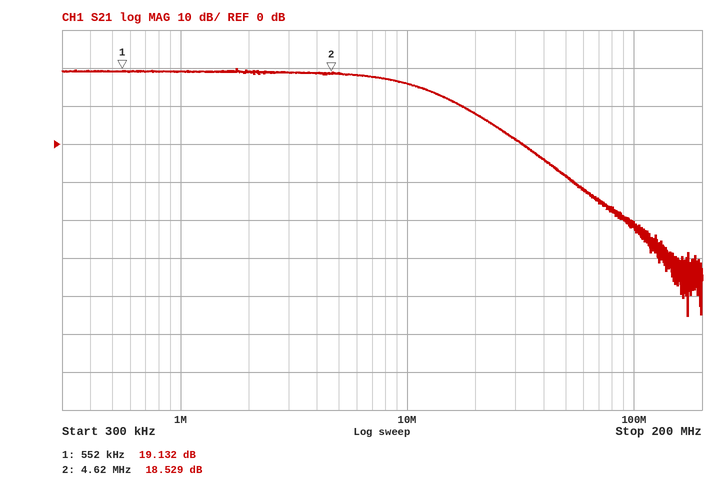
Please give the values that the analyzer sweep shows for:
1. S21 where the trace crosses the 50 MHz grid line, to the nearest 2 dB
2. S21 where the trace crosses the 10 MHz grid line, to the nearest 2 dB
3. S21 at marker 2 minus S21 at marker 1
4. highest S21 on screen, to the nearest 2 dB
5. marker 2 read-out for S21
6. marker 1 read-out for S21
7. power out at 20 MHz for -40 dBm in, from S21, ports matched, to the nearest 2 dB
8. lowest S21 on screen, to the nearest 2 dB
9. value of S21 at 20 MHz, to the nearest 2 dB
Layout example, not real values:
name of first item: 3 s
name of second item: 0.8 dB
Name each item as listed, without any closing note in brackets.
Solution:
S21 where the trace crosses the 50 MHz grid line, to the nearest 2 dB: -8 dB
S21 where the trace crosses the 10 MHz grid line, to the nearest 2 dB: 16 dB
S21 at marker 2 minus S21 at marker 1: -0.603 dB
highest S21 on screen, to the nearest 2 dB: 20 dB
marker 2 read-out for S21: 18.529 dB
marker 1 read-out for S21: 19.132 dB
power out at 20 MHz for -40 dBm in, from S21, ports matched, to the nearest 2 dB: -32 dBm
lowest S21 on screen, to the nearest 2 dB: -46 dB
value of S21 at 20 MHz, to the nearest 2 dB: 8 dB
